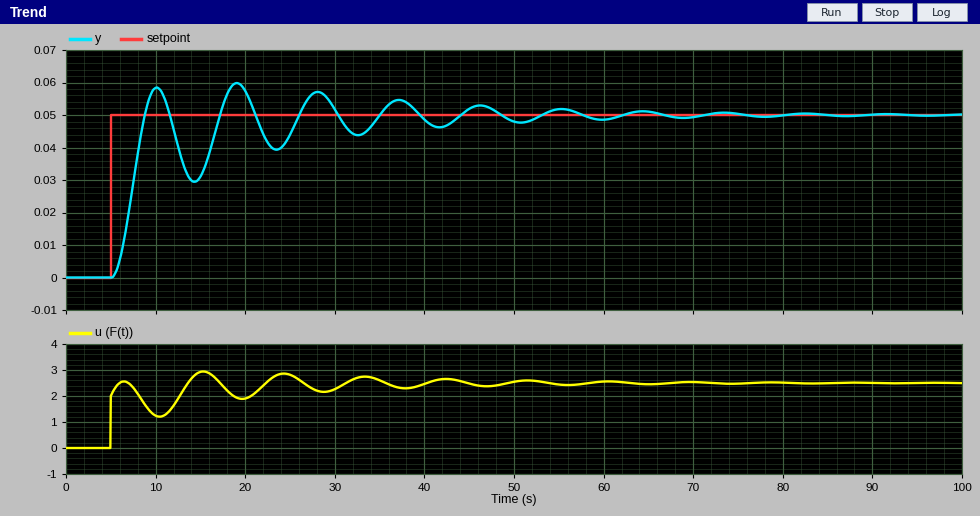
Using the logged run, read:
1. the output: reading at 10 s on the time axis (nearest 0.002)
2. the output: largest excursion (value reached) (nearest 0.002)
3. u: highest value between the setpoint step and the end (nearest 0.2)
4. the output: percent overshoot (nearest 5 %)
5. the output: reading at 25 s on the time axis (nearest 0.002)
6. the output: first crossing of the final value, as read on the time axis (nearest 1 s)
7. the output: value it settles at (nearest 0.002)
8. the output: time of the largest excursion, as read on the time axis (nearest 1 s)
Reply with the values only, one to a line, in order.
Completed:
0.058
0.060
3.0
20 %
0.044
9 s
0.050
19 s
